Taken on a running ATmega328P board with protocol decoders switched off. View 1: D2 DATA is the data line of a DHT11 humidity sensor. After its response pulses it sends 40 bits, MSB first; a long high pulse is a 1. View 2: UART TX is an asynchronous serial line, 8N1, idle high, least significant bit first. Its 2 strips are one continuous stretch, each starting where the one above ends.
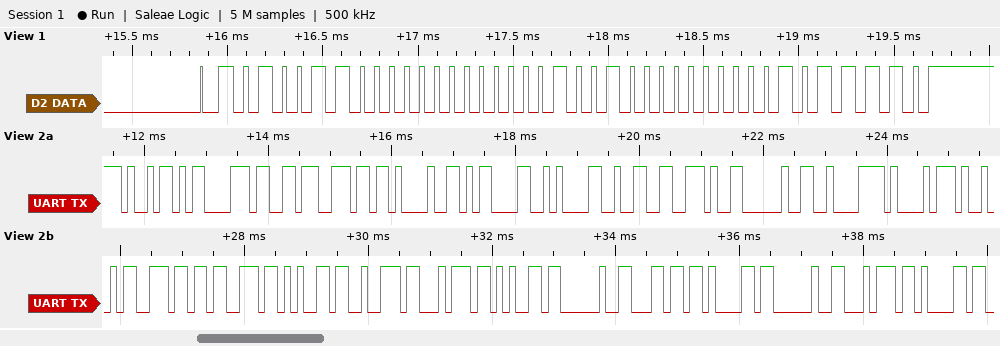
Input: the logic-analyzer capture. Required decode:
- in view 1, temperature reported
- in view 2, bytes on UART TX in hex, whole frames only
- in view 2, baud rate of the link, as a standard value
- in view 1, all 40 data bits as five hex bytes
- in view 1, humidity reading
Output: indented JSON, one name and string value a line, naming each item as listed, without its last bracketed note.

{
  "in view 1, temperature reported": "18.0 °C",
  "in view 2, bytes on UART TX in hex, whole frames only": "69 C3 B3 6E 21 0D 0A 32 2E 20 C2 A1 49 6E 73 65 72 74 65 20 6C 61 20 74 61",
  "in view 2, baud rate of the link, as a standard value": "9600 baud",
  "in view 1, all 40 data bits as five hex bytes": "4C 00 12 00 5E",
  "in view 1, humidity reading": "76 %"
}
